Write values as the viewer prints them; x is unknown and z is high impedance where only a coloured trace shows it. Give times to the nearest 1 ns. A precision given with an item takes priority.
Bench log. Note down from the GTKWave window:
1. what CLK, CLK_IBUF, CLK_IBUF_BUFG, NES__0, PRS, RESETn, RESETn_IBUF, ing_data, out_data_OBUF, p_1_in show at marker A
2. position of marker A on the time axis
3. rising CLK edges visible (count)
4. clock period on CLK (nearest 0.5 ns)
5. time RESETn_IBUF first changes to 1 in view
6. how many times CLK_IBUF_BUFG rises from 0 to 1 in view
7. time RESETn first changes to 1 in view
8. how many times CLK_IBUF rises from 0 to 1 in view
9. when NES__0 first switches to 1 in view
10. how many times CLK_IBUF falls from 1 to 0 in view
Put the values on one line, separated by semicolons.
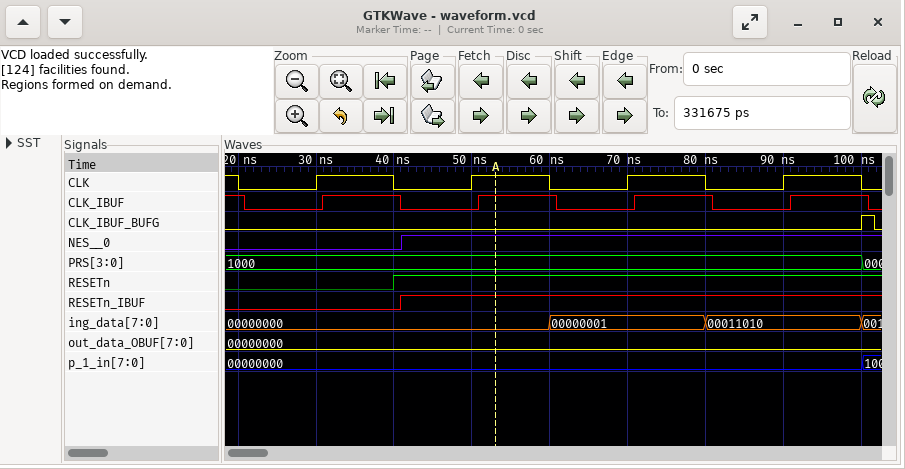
CLK=1, CLK_IBUF=1, CLK_IBUF_BUFG=0, NES__0=1, PRS=1000, RESETn=1, RESETn_IBUF=1, ing_data=00000000, out_data_OBUF=00000000, p_1_in=00000000; 53 ns; 4; 20 ns; 41 ns; 1; 40 ns; 4; 41 ns; 5
